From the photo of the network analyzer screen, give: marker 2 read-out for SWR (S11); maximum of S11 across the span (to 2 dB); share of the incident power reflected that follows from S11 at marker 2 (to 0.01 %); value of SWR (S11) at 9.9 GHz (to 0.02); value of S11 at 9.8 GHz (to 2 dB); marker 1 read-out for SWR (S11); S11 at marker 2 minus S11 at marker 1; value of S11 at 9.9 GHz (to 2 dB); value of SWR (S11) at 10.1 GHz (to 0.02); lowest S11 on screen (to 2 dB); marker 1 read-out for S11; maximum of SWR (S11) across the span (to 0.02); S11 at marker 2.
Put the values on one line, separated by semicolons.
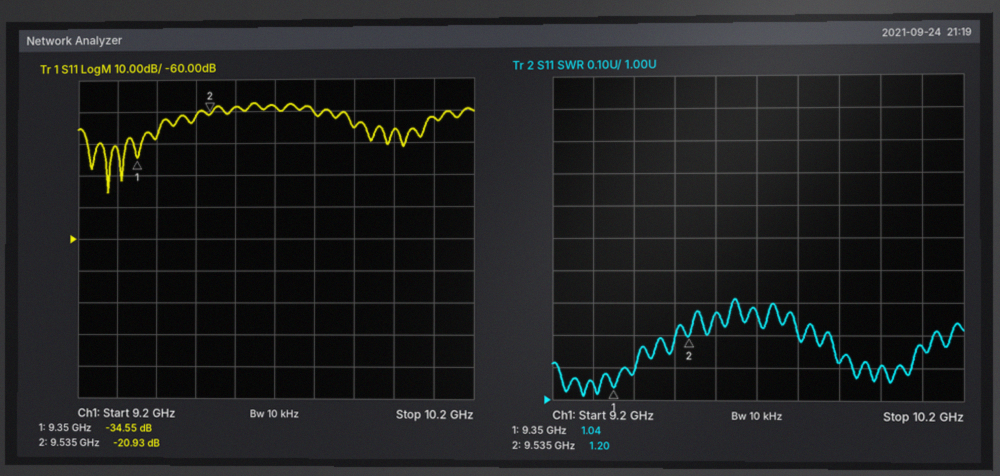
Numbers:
1.20; -18 dB; 0.81 %; 1.12; -20 dB; 1.04; 13.62 dB; -26 dB; 1.16; -46 dB; -34.55 dB; 1.32; -20.93 dB
